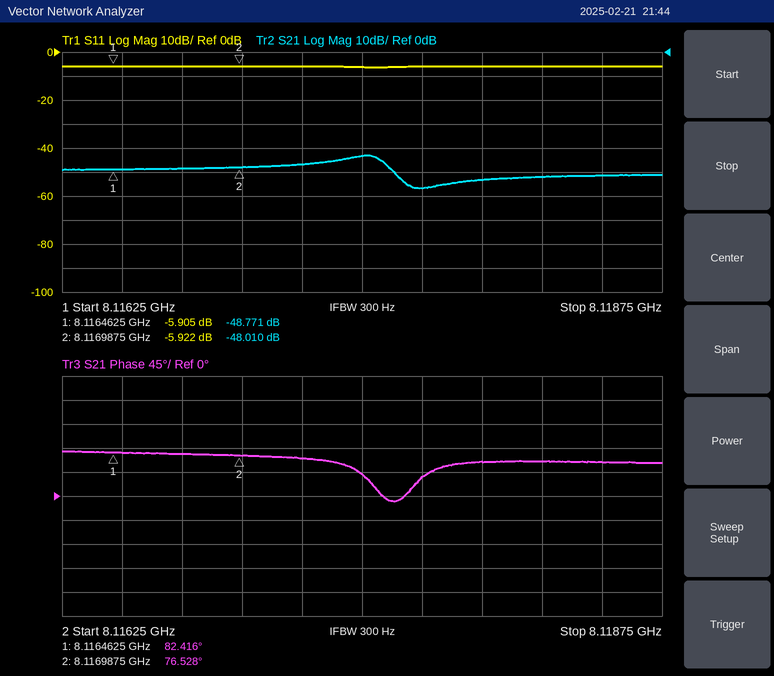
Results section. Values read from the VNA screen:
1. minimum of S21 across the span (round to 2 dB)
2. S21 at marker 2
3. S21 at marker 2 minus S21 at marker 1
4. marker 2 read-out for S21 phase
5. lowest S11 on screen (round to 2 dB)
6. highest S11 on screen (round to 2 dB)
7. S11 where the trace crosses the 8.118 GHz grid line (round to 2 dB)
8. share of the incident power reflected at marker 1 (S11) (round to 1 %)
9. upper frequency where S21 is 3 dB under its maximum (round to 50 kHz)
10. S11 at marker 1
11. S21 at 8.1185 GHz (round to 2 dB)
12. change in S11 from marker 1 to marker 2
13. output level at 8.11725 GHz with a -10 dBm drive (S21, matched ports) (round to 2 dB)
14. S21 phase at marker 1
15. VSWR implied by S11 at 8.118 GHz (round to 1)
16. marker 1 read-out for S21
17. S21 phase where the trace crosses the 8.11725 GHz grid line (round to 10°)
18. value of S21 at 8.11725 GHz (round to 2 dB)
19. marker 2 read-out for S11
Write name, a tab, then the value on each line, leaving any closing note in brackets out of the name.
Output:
minimum of S21 across the span	-56 dB
S21 at marker 2	-48.010 dB
S21 at marker 2 minus S21 at marker 1	0.761 dB
marker 2 read-out for S21 phase	76.528°
lowest S11 on screen	-6 dB
highest S11 on screen	-6 dB
S11 where the trace crosses the 8.118 GHz grid line	-6 dB
share of the incident power reflected at marker 1 (S11)	26 %
upper frequency where S21 is 3 dB under its maximum	8.11760 GHz
S11 at marker 1	-5.905 dB
S21 at 8.1185 GHz	-52 dB
change in S11 from marker 1 to marker 2	-0.017 dB
output level at 8.11725 GHz with a -10 dBm drive (S21, matched ports)	-56 dBm
S21 phase at marker 1	82.416°
VSWR implied by S11 at 8.118 GHz	3
marker 1 read-out for S21	-48.771 dB
S21 phase where the trace crosses the 8.11725 GHz grid line	70°
value of S21 at 8.11725 GHz	-46 dB
marker 2 read-out for S11	-5.922 dB
